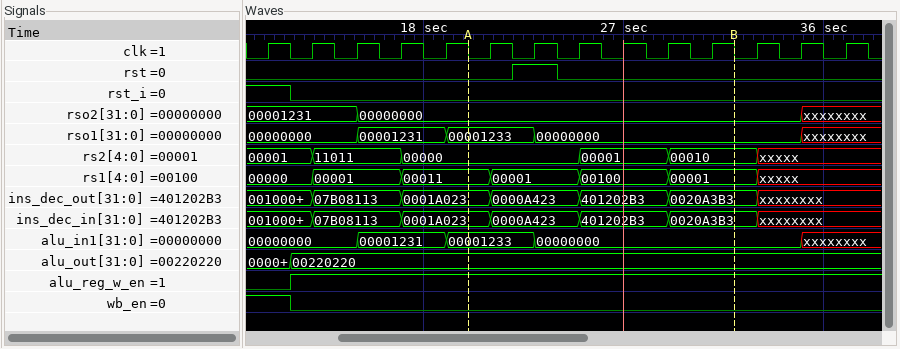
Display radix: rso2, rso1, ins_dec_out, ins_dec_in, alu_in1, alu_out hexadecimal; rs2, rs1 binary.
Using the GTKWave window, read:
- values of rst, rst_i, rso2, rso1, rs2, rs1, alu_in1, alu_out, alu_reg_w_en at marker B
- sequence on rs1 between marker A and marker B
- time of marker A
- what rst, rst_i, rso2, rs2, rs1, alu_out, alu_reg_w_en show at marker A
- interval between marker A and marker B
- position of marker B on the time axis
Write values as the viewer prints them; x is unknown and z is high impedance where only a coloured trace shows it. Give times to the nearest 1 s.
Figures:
rst=0, rst_i=0, rso2=00000000, rso1=00000000, rs2=00010, rs1=00001, alu_in1=00000000, alu_out=00220220, alu_reg_w_en=1
00011, 00001, 00100, 00001
20 s
rst=0, rst_i=0, rso2=00000000, rs2=00000, rs1=00011, alu_out=00220220, alu_reg_w_en=1
12 s
32 s
